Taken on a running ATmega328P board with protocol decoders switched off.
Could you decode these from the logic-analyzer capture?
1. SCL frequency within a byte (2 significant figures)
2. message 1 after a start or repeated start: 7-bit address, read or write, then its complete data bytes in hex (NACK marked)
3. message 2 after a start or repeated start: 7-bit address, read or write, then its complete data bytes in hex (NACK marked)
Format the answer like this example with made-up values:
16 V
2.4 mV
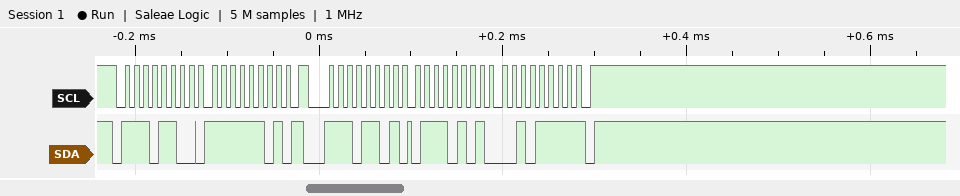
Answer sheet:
100 kHz
0x76 write: FD
0x76 read: 75 2F NACK
